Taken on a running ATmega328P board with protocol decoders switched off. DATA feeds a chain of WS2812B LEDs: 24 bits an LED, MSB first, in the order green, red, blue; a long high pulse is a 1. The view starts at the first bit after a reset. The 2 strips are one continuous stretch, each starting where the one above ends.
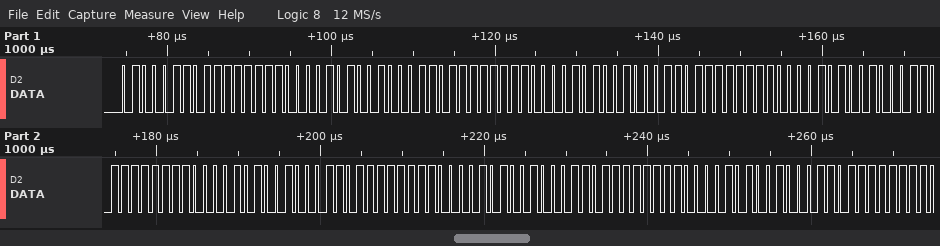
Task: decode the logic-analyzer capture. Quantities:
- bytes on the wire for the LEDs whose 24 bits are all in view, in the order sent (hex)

46 FF 0A 46 FF 0A 46 FF 0A 46 FF 0A 46 FF 0A 46 FF 0A
